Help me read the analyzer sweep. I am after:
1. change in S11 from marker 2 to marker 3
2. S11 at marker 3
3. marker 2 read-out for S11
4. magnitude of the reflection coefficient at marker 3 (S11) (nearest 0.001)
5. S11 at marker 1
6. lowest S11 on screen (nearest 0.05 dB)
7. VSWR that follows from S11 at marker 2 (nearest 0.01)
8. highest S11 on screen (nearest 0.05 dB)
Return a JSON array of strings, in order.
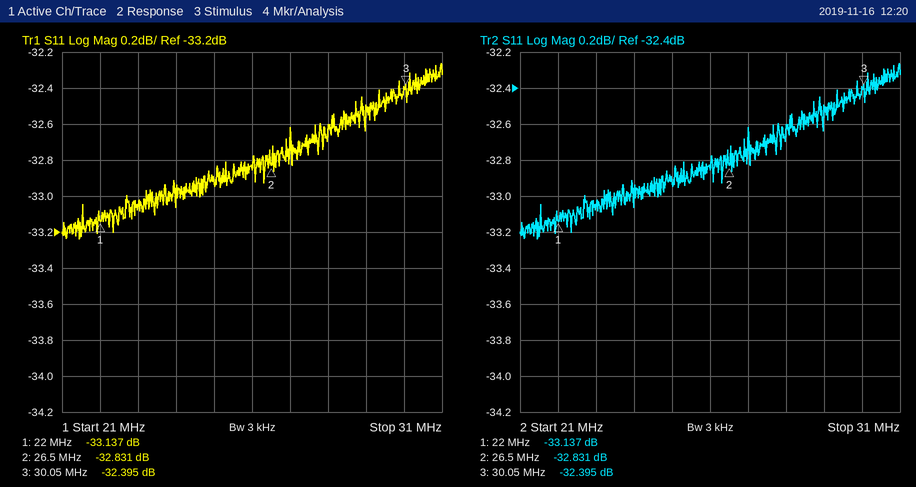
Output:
["0.436 dB", "-32.395 dB", "-32.831 dB", "0.024", "-33.137 dB", "-33.25 dB", "1.05", "-32.25 dB"]
